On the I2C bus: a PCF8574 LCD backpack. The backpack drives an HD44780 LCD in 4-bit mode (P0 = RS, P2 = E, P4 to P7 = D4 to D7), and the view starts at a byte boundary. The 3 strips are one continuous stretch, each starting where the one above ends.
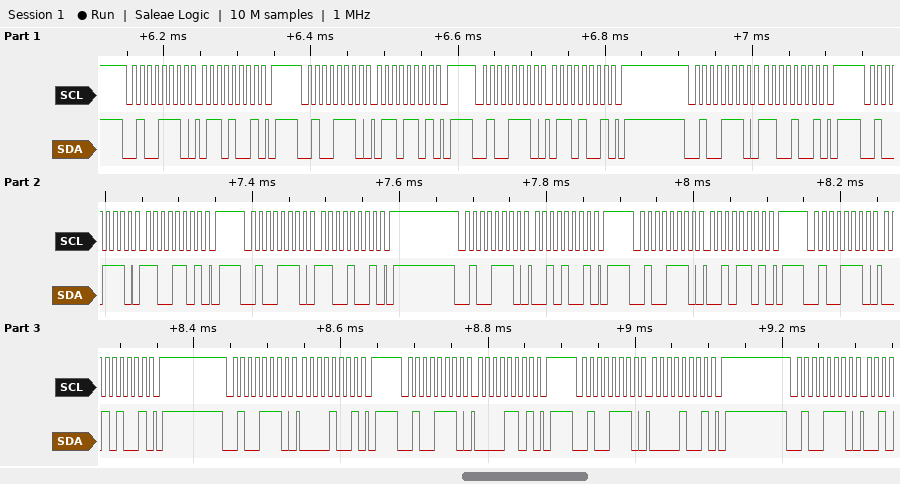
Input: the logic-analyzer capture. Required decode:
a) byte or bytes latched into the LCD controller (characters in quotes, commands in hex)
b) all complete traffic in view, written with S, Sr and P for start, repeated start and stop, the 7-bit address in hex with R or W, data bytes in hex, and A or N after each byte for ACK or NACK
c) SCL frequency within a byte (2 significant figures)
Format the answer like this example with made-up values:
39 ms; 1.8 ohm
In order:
'l' ' '; S 27W A 69 A P S 27W A 6D A P S 27W A 69 A P S 27W A C9 A P S 27W A CD A P S 27W A C9 A P S 27W A 29 A P S 27W A 2D A P S 27W A 29 A P S 27W A 09 A P S 27W A 0D A P S 27W A 09 A P S 27W A; 100 kHz
